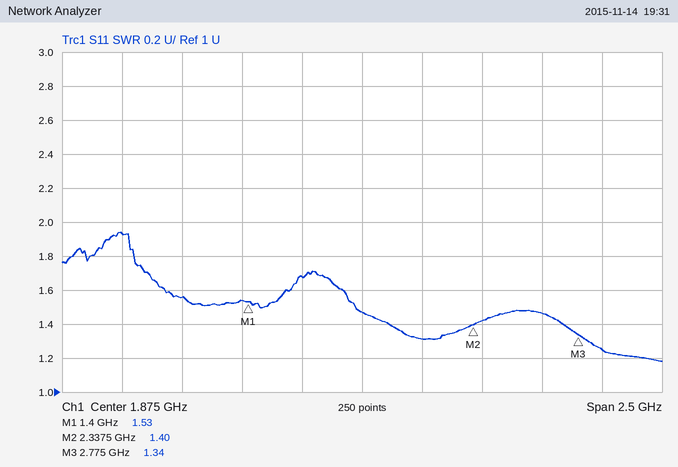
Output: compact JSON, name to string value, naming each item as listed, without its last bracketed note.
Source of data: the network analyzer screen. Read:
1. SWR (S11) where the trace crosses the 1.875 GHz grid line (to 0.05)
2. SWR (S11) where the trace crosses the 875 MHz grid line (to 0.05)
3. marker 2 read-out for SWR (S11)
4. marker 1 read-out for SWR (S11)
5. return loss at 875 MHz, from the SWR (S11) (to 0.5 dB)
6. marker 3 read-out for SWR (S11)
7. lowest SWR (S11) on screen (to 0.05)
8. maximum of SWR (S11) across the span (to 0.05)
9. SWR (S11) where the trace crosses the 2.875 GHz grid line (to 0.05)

{"SWR (S11) where the trace crosses the 1.875 GHz grid line": "1.45", "SWR (S11) where the trace crosses the 875 MHz grid line": "1.95", "marker 2 read-out for SWR": "1.40", "marker 1 read-out for SWR": "1.53", "return loss at 875 MHz, from the SWR (S11)": "10.0 dB", "marker 3 read-out for SWR": "1.34", "lowest SWR (S11) on screen": "1.20", "maximum of SWR (S11) across the span": "1.95", "SWR (S11) where the trace crosses the 2.875 GHz grid line": "1.25"}
